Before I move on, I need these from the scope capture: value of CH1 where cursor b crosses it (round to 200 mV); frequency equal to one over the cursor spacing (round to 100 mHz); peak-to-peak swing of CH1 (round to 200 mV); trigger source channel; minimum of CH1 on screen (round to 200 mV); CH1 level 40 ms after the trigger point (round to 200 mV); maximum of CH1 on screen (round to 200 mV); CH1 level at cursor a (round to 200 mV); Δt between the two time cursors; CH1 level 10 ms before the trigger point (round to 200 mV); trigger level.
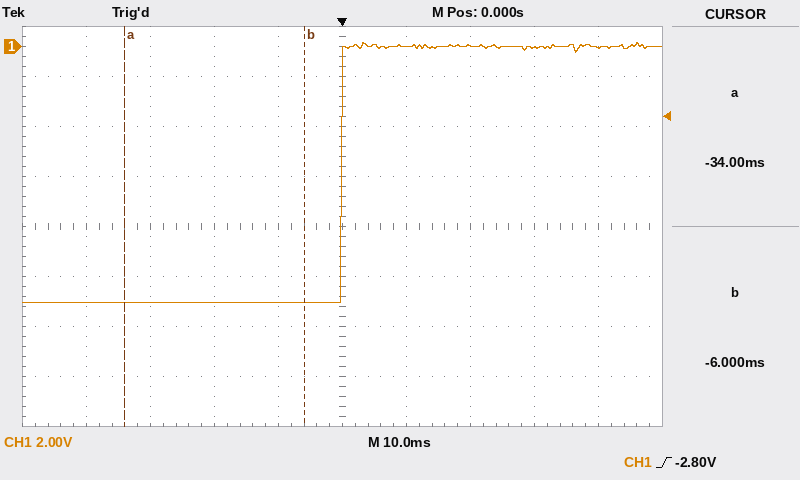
-10.2 V
35.7 Hz
10.4 V
CH1
-10.2 V
0.0 V
200 mV
-10.2 V
28 ms
-10.2 V
-2.80 V
